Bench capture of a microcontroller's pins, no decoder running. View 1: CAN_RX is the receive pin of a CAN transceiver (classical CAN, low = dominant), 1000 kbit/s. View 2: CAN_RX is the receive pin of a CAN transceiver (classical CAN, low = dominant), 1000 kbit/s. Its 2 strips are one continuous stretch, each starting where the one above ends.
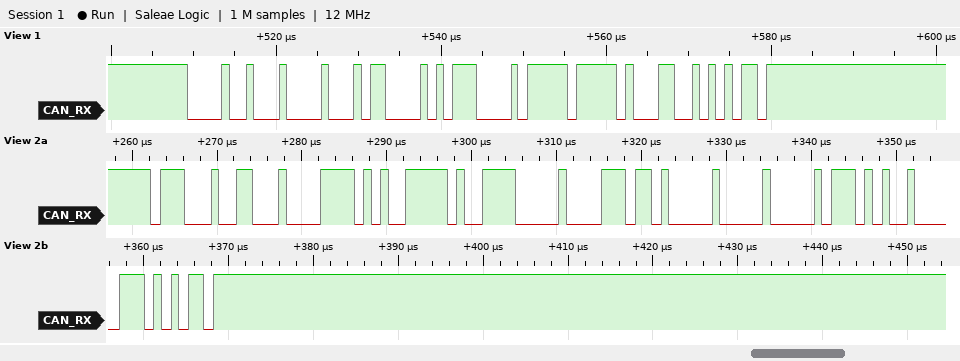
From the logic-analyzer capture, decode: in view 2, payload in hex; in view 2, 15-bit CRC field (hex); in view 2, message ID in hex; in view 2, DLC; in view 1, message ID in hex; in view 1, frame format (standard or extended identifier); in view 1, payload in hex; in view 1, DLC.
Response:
7A 9F 9E 00 ED 00 00 EA
0x20D5
0x713
8
0x091
standard
58 57 0B FF
4
